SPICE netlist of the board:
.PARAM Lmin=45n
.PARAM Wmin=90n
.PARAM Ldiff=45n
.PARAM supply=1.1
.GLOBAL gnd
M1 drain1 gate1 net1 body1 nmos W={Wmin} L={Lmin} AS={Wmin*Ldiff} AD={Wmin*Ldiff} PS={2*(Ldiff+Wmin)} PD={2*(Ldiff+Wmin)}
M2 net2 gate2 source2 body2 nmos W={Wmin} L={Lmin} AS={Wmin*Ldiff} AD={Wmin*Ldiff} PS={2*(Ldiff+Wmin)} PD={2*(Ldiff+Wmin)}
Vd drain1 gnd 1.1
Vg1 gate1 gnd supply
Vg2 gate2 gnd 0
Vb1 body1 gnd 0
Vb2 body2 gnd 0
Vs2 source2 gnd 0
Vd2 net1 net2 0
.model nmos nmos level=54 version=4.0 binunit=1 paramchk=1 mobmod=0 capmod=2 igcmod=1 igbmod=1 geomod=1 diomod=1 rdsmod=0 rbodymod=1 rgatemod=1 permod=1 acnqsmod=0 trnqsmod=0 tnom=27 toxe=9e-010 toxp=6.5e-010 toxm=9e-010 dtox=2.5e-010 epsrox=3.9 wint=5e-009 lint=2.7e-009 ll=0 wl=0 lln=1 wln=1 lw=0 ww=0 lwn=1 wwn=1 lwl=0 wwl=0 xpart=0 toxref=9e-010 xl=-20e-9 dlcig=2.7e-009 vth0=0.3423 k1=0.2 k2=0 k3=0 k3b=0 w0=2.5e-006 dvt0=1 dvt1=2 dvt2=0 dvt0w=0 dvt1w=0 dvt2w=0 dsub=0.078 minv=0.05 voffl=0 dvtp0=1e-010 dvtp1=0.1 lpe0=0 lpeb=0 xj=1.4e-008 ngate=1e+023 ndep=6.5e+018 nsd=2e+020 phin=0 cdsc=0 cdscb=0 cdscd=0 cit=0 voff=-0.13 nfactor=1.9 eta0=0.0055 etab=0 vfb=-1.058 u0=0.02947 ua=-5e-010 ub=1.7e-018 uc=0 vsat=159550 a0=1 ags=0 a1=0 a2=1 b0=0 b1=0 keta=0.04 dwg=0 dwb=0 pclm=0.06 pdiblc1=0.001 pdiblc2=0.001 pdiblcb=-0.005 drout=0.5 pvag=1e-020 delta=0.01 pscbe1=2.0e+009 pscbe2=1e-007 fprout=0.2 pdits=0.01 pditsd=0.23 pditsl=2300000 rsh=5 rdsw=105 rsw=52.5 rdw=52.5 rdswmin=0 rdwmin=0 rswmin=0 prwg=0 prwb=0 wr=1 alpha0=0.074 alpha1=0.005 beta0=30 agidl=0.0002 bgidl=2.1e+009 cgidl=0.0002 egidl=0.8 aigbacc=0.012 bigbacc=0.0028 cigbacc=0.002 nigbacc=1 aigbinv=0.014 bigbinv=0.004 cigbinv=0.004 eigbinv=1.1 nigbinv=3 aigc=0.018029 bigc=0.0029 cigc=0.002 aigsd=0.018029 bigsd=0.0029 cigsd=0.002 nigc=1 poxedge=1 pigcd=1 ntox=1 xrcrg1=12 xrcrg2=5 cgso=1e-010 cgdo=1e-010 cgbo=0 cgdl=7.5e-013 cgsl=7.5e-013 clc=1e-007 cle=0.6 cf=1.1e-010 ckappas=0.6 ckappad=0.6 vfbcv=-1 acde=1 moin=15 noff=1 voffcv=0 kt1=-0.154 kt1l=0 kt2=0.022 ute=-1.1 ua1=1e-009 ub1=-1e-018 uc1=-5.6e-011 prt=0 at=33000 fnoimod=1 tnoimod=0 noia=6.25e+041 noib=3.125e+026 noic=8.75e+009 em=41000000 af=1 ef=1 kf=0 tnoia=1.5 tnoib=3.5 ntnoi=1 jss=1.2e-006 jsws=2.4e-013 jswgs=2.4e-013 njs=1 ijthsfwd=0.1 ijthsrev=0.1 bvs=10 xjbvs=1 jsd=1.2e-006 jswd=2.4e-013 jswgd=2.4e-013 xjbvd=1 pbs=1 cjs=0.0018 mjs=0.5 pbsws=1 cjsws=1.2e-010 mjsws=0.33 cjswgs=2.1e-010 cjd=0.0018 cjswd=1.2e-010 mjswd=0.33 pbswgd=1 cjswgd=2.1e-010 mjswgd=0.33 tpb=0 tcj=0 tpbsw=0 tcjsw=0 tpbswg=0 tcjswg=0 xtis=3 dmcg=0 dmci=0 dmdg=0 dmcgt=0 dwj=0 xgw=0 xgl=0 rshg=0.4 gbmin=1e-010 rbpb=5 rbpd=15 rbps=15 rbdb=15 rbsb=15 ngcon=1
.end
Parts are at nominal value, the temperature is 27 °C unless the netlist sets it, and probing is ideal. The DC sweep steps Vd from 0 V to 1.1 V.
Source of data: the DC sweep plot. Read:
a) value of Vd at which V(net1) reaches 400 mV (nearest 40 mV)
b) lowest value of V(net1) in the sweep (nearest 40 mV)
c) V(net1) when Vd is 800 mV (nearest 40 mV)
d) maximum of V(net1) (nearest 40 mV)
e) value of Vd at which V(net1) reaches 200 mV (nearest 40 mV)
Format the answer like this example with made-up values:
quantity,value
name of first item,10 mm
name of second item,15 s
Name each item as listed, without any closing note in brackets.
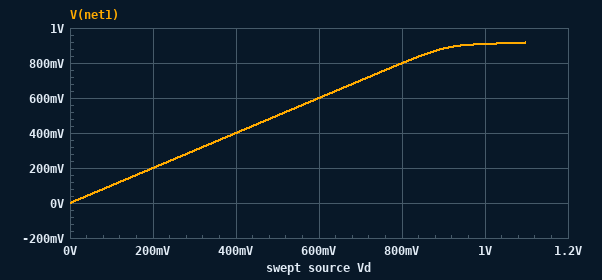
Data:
quantity,value
value of Vd at which V(net1) reaches 400 mV,400 mV
lowest value of V(net1) in the sweep,0 V
V(net1) when Vd is 800 mV,800 mV
maximum of V(net1),920 mV
value of Vd at which V(net1) reaches 200 mV,200 mV
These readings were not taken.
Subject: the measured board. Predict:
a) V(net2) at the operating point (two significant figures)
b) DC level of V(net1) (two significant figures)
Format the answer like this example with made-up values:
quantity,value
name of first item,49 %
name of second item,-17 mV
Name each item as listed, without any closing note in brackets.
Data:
quantity,value
V(net2) at the operating point,920 mV
DC level of V(net1),920 mV
